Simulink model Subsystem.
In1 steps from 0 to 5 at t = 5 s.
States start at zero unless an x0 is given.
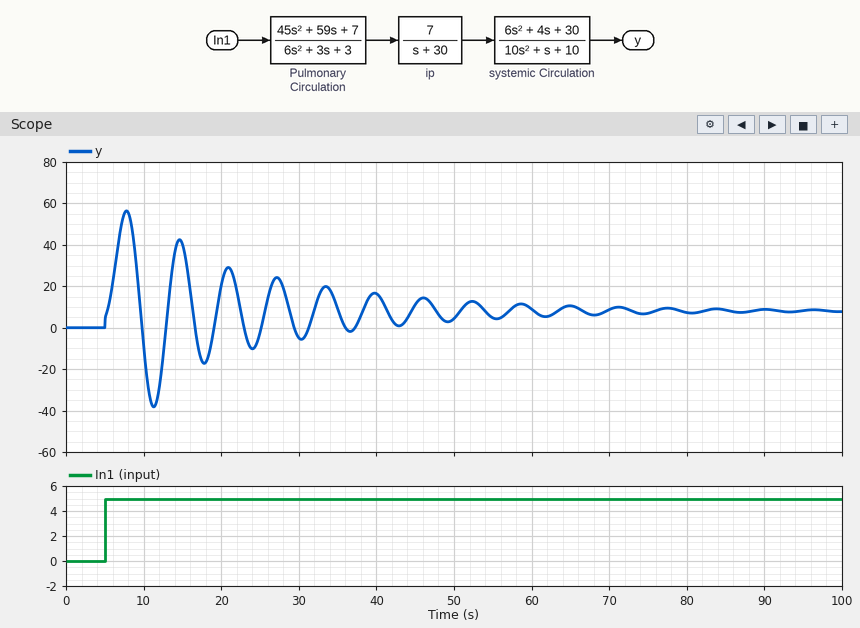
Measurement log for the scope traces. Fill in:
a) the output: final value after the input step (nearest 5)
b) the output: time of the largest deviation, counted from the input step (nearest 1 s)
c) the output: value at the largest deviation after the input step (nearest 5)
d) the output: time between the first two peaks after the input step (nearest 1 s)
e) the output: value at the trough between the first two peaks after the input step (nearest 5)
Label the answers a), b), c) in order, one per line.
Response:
a) 10
b) 3 s
c) 55
d) 7 s
e) -40
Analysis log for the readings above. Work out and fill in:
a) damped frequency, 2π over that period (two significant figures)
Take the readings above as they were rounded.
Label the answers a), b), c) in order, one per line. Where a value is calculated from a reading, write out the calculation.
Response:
a) 2π / 7 = 0.90 rad/s
